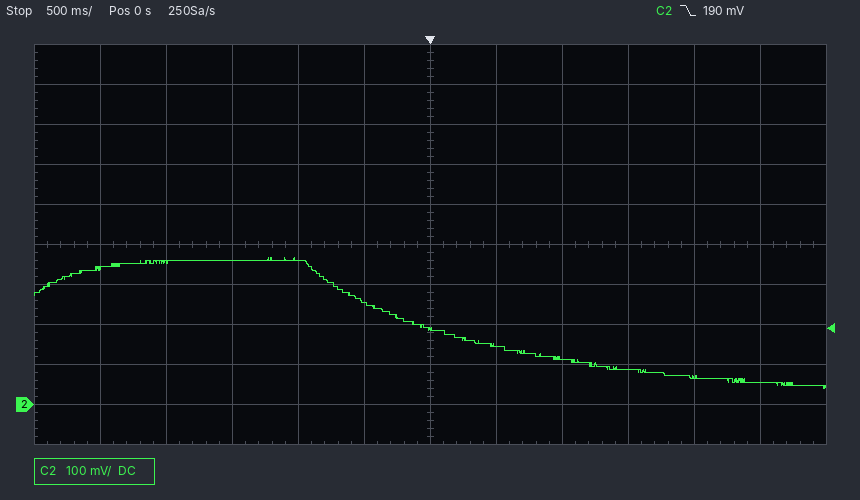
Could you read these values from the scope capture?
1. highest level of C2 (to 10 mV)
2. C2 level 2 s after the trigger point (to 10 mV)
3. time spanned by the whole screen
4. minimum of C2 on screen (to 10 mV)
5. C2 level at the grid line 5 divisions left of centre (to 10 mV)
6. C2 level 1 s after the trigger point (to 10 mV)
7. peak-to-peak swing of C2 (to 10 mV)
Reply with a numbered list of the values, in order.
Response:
1. 370 mV
2. 70 mV
3. 6 s
4. 40 mV
5. 340 mV
6. 120 mV
7. 330 mV
